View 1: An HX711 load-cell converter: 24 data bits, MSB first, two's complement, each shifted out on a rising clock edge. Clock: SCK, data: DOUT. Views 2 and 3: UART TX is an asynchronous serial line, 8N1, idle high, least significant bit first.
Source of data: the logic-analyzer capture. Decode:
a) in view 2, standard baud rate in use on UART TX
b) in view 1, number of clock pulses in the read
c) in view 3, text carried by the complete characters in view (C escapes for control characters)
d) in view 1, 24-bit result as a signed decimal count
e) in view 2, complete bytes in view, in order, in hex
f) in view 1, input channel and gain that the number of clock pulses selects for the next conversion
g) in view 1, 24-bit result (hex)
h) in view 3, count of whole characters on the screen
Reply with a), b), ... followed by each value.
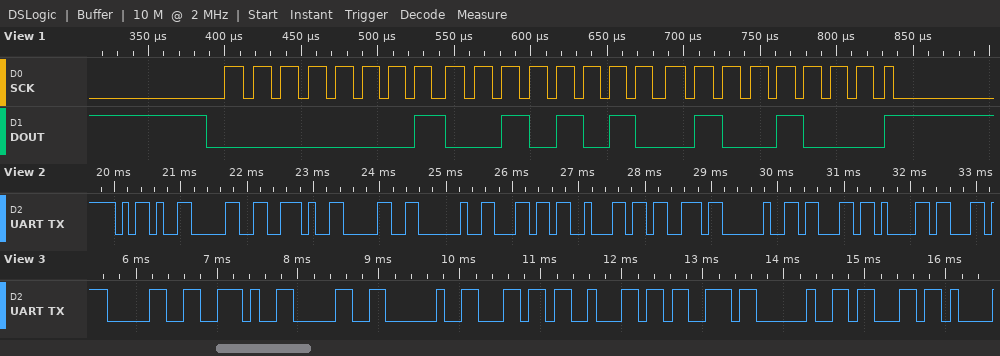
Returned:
a) 9600 baud
b) 25
c) "0.0 lbs c"
d) 76360
e) 2D 30 2E 30 20 6C 62 73 20 63 61
f) channel A, gain 128
g) 0x012A48
h) 9
